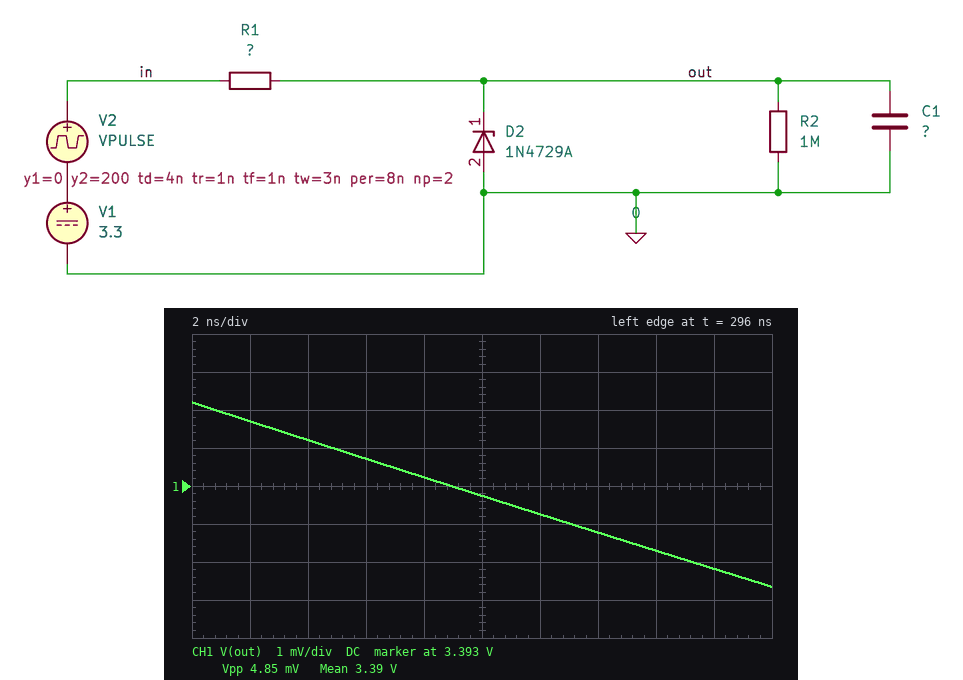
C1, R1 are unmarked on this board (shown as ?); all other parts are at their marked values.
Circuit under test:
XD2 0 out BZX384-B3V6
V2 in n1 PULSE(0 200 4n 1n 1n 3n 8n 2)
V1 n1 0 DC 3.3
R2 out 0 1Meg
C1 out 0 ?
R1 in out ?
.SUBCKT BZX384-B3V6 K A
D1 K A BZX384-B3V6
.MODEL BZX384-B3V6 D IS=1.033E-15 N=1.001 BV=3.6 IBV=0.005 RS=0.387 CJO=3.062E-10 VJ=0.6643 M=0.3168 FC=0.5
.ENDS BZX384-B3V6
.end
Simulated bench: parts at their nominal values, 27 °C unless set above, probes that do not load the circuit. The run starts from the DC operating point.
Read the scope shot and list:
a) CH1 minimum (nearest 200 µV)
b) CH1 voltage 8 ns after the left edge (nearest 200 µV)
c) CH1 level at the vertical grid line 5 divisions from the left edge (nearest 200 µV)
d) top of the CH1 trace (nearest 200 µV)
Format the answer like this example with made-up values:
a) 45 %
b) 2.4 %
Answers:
a) 3.3904 V
b) 3.3932 V
c) 3.3928 V
d) 3.3952 V
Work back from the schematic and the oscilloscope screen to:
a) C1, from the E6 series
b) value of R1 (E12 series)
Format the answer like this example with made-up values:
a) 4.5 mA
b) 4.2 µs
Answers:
a) 22 pF
b) 2.2 kΩ
